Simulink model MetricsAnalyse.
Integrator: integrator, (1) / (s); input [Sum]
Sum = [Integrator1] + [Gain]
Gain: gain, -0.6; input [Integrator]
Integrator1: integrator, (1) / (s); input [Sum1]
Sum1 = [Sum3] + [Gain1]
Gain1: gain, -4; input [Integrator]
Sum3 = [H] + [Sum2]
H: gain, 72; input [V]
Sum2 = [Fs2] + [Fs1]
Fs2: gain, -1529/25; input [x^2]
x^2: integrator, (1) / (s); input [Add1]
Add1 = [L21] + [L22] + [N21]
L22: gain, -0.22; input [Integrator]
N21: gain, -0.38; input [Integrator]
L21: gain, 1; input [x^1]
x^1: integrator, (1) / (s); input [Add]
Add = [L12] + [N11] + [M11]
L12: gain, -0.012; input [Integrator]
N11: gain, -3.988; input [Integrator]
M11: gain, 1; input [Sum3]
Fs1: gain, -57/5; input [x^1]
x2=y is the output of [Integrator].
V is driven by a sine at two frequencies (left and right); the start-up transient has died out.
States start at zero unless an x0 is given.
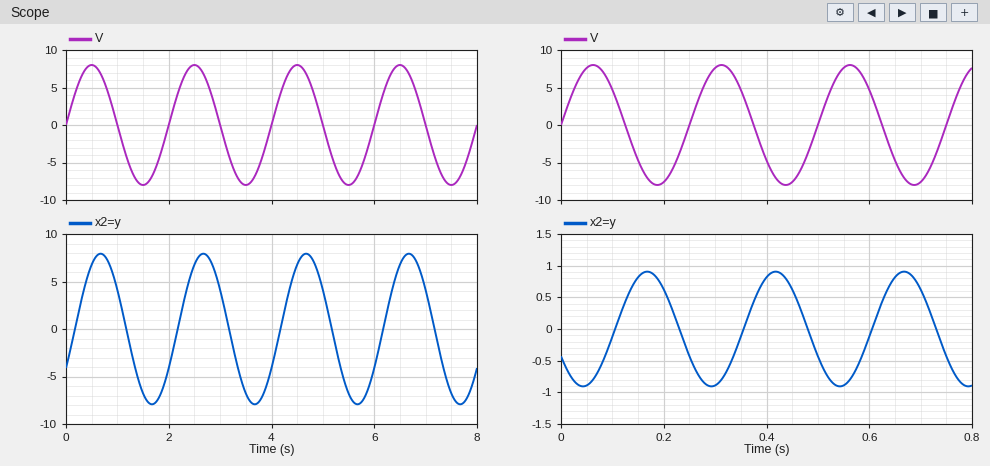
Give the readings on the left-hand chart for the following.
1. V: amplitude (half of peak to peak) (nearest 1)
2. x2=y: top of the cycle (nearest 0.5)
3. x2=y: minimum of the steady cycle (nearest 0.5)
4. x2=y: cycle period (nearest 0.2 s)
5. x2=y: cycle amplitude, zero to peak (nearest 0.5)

8
8.0
-8.0
2.0 s
8.0
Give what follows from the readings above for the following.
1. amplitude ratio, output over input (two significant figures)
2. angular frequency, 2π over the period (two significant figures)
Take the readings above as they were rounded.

1.0
3.1 rad/s
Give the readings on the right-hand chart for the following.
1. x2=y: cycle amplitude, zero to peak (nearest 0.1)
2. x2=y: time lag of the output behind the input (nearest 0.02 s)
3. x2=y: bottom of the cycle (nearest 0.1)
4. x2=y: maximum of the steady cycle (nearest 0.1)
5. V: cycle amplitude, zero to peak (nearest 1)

0.9
0.10 s
-0.9
0.9
8
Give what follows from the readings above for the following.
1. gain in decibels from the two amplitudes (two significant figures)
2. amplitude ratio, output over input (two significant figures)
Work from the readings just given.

-19 dB
0.11
